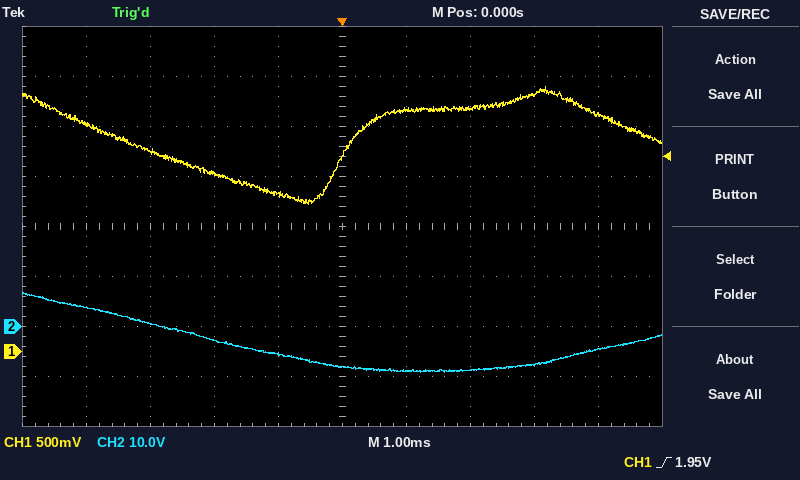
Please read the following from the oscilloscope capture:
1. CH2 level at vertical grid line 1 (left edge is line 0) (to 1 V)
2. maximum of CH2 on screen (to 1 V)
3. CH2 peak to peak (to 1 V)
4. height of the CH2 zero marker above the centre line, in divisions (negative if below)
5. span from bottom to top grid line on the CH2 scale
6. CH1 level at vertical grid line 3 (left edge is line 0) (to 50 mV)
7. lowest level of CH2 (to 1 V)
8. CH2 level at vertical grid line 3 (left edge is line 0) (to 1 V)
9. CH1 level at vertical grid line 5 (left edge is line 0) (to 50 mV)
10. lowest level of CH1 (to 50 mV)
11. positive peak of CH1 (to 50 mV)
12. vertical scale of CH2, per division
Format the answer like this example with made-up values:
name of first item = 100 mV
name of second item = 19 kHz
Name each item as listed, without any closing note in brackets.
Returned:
CH2 level at vertical grid line 1 (left edge is line 0) = 4 V
maximum of CH2 on screen = 7 V
CH2 peak to peak = 16 V
height of the CH2 zero marker above the centre line, in divisions = -2.0 div
span from bottom to top grid line on the CH2 scale = 80 V
CH1 level at vertical grid line 3 (left edge is line 0) = 1.80 V
lowest level of CH2 = -9 V
CH2 level at vertical grid line 3 (left edge is line 0) = -3 V
CH1 level at vertical grid line 5 (left edge is line 0) = 1.95 V
lowest level of CH1 = 1.45 V
positive peak of CH1 = 2.65 V
vertical scale of CH2, per division = 10 V
